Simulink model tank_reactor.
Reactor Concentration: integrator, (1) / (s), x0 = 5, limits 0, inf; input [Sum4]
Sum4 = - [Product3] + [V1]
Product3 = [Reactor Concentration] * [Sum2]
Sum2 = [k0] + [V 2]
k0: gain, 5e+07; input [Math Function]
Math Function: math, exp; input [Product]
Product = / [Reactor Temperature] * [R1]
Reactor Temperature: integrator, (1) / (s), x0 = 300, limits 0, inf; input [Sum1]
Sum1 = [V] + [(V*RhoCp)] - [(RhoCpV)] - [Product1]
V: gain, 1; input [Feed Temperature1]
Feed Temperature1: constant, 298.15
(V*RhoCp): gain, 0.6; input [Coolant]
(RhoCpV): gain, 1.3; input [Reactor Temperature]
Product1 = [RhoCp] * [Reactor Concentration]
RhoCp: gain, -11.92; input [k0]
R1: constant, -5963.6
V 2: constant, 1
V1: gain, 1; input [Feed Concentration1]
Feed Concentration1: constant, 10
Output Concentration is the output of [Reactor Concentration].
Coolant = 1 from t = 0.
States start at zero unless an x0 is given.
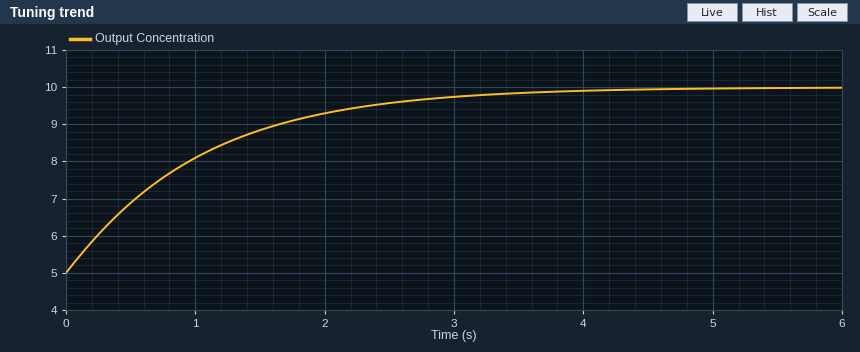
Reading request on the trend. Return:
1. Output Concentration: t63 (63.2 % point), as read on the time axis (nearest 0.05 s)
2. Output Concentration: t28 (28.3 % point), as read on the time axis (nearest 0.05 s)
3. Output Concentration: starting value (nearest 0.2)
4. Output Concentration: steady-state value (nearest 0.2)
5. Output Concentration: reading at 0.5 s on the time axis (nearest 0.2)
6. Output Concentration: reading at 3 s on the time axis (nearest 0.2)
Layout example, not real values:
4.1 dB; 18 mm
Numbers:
1.05 s; 0.35 s; 5.0; 10.0; 6.8; 9.8
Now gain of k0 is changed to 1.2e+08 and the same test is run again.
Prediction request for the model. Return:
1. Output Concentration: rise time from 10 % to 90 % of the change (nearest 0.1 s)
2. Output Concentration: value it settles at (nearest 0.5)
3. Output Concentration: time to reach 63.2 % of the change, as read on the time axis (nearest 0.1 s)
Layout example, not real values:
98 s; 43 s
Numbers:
2.3 s; 10.0; 1.1 s
